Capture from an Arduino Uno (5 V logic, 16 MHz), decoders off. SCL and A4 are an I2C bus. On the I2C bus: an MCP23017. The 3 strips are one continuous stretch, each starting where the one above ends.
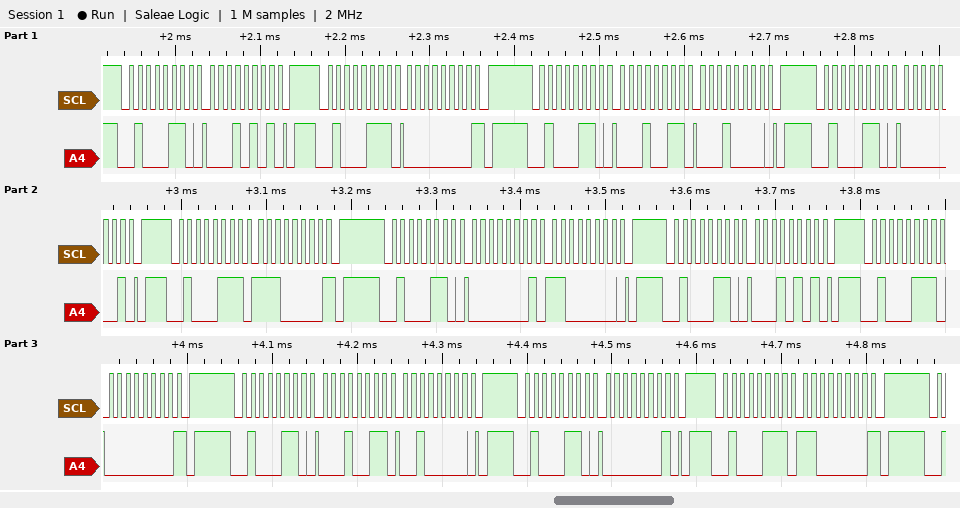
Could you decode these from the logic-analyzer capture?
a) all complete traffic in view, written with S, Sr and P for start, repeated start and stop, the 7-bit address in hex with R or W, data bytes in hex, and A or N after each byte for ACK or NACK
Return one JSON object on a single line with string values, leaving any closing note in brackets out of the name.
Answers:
{"all complete traffic in view, written with S, Sr and P for start, repeated start and stop, the 7-bit address in hex with R or W, data bytes in hex, and A or N after each byte for ACK or NACK": "S 23W A 15 A P S 23R A 00 N P S 23W A 13 A 10 A P S 23W A 01 A P S 23R A E0 N P S 23W A 01 A C0 A P S 23W A 15 A P S 23R A 00 N P S 23W A 13 A 20 A P S 23W A 01 A P S 23R A C0 N P"}
